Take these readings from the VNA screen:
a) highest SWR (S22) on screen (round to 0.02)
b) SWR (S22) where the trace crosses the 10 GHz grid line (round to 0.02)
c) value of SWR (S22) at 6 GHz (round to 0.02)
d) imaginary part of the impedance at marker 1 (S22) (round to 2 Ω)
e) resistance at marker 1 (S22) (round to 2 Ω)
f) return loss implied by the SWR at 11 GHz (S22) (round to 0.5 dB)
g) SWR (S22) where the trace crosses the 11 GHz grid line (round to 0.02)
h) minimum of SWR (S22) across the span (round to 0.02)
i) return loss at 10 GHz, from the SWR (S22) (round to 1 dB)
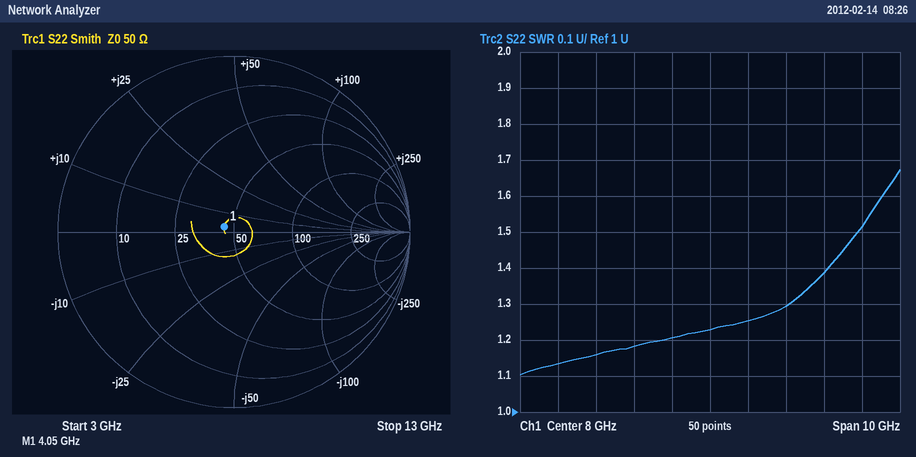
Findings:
1.68
1.30
1.18
+2 Ω
44 Ω
16.0 dB
1.38
1.10
18 dB
